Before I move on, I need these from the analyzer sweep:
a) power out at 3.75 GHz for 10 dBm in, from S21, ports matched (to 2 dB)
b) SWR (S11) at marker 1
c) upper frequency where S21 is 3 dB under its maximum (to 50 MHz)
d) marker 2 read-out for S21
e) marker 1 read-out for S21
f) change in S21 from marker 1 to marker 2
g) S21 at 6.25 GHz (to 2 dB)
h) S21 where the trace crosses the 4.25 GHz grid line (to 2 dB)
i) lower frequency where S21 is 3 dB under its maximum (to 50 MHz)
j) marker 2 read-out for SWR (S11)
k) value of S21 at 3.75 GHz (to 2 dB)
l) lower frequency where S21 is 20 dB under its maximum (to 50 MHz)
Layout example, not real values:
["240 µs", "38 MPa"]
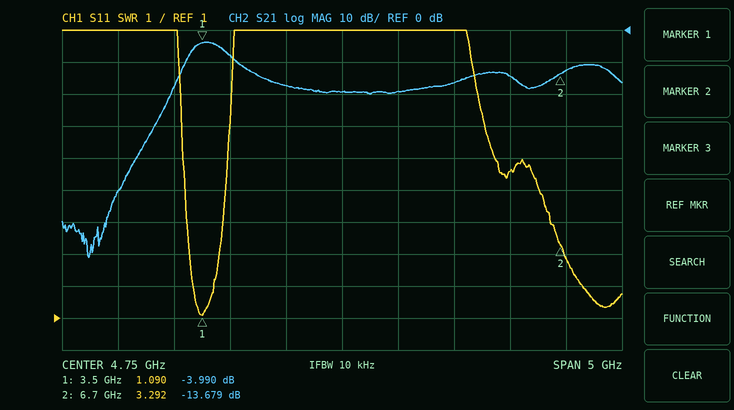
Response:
["2 dBm", "1.090", "3.70 GHz", "-13.679 dB", "-3.990 dB", "-9.689 dB", "-14 dB", "-18 dB", "3.40 GHz", "3.292", "-8 dB", "3.15 GHz"]
